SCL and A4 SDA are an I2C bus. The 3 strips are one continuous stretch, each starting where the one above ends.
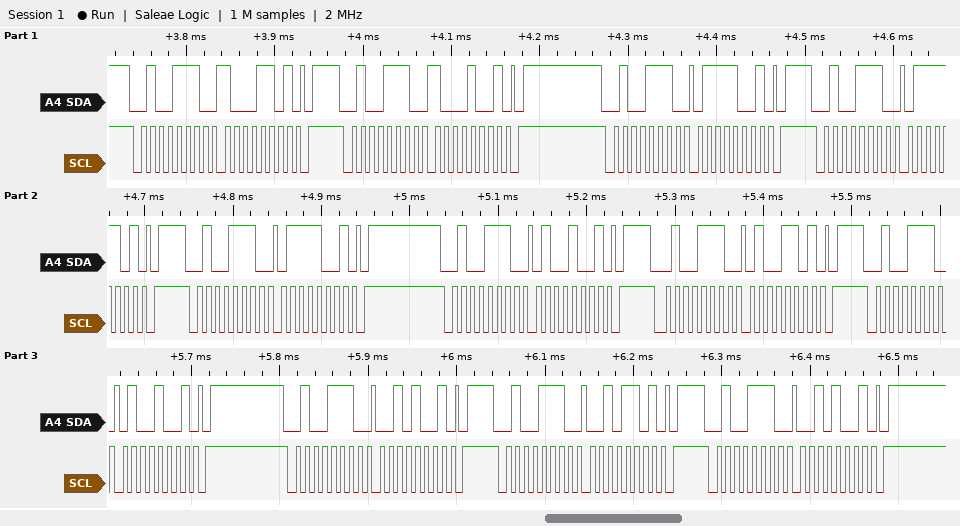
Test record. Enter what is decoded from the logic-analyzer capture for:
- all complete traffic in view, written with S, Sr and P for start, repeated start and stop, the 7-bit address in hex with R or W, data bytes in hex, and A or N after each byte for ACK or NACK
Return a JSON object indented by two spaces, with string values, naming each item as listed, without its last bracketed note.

{
  "all complete traffic in view, written with S, Sr and P for start, repeated start and stop, the 7-bit address in hex with R or W, data bytes in hex, and A or N after each byte for ACK or NACK": "S 27W A 8D A P S 27W A 89 A P S 27W A 79 A P S 27W A 7D A P S 27W A 79 A P S 27W A 49 A P S 27W A 4D A P S 27W A 49 A P S 27W A 29 A P S 27W A 2D A P S 27W A 29 A P"
}
